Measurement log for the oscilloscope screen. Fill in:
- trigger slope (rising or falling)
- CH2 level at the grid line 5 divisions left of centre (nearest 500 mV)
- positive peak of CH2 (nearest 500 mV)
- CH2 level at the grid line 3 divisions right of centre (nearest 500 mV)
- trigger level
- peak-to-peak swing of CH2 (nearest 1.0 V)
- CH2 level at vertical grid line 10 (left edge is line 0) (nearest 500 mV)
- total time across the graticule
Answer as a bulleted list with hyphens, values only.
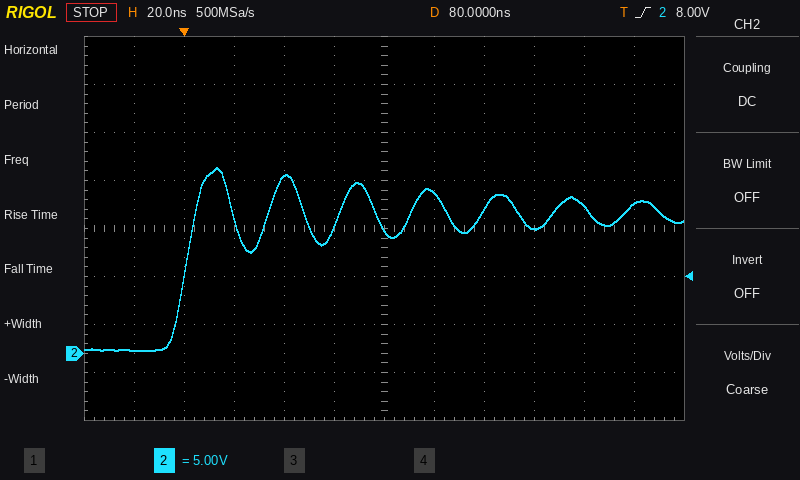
- rising
- 500 mV
- 19.5 V
- 13.0 V
- 8.00 V
- 19.0 V
- 15.5 V
- 240 ns
